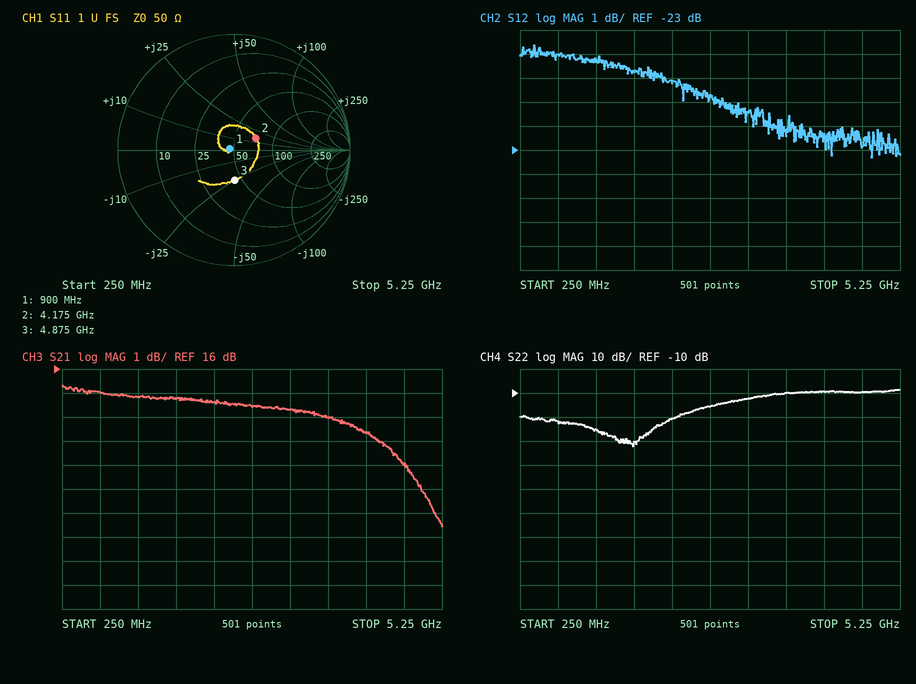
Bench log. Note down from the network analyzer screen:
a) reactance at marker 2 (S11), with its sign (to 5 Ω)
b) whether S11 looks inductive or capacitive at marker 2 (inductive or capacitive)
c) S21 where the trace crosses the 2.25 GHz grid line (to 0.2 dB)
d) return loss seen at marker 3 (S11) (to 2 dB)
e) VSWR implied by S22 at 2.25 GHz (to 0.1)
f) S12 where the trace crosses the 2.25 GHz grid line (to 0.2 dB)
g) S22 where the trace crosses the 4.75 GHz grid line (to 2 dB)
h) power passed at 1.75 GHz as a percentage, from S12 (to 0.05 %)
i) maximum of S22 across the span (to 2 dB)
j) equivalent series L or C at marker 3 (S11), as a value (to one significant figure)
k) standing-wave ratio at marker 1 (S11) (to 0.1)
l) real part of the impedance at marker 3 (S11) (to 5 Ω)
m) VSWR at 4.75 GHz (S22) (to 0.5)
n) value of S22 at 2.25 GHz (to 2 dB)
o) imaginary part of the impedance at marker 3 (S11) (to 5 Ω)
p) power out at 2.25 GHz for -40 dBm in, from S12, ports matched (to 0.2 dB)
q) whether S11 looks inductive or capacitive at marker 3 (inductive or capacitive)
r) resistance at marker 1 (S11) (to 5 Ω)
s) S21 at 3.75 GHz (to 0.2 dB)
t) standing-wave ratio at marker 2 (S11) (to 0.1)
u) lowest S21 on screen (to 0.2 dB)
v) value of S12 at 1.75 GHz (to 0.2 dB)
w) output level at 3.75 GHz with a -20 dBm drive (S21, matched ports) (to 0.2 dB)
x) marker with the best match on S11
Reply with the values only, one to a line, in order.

+15 Ω
inductive
14.6 dB
12 dB
1.2
-20.2 dB
-10 dB
1.05 %
-8 dB
1 pF
1.1
45 Ω
2.0
-20 dB
-25 Ω
-60.2 dBm
capacitive
45 Ω
14.0 dB
1.5
9.4 dB
-19.8 dB
-6.0 dBm
marker 1
